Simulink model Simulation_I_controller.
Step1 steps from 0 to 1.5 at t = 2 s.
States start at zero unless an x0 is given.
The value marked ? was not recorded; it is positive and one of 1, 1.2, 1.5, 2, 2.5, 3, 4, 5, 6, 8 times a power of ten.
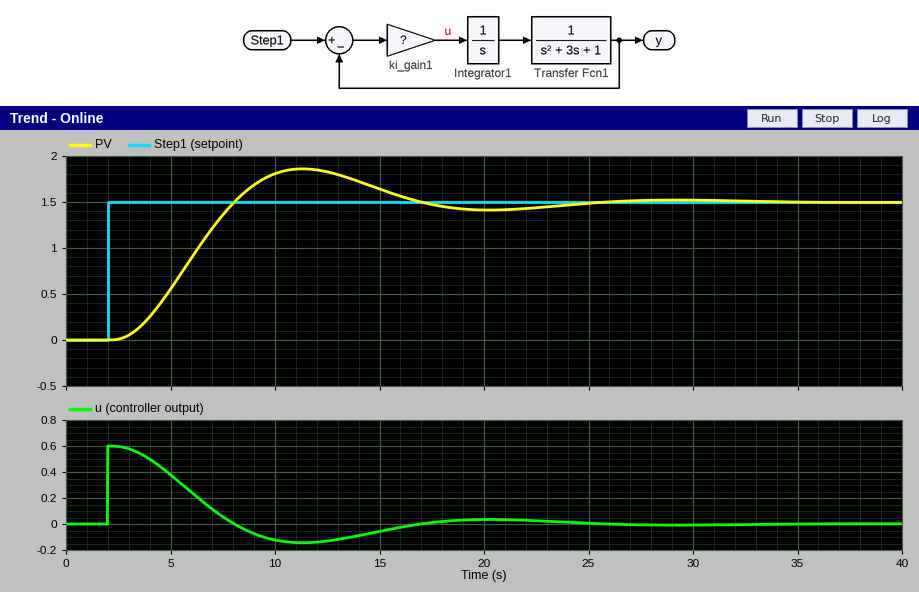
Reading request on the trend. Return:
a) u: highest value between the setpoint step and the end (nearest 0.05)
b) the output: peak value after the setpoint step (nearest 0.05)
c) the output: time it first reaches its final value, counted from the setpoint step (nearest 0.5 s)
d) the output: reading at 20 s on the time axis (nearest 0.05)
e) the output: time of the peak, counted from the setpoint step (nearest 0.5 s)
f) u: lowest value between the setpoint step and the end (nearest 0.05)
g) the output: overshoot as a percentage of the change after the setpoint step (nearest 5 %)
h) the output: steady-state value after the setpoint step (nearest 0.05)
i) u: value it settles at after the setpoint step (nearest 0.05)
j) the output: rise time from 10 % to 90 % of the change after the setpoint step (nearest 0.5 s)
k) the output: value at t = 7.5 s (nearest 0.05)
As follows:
0.60
1.85
6.0 s
1.40
9.5 s
-0.15
25 %
1.50
0.00
4.0 s
1.35
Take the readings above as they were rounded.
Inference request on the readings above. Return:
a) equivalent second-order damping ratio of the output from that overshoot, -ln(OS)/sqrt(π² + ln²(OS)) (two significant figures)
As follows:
0.40
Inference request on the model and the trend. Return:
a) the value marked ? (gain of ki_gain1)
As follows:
0.4
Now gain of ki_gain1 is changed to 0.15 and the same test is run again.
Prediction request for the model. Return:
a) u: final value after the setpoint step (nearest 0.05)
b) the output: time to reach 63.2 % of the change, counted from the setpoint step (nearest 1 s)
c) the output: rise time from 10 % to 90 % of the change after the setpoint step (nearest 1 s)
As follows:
0.00
8 s
10 s
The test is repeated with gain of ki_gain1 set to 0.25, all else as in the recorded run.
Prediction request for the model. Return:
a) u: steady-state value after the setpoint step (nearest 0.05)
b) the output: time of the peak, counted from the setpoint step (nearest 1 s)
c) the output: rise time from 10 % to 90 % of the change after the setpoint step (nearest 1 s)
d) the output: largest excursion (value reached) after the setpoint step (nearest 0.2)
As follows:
0.00
13 s
6 s
1.6
